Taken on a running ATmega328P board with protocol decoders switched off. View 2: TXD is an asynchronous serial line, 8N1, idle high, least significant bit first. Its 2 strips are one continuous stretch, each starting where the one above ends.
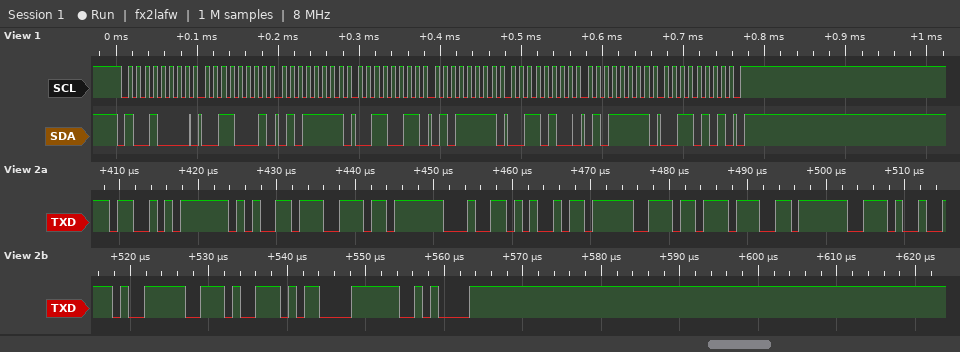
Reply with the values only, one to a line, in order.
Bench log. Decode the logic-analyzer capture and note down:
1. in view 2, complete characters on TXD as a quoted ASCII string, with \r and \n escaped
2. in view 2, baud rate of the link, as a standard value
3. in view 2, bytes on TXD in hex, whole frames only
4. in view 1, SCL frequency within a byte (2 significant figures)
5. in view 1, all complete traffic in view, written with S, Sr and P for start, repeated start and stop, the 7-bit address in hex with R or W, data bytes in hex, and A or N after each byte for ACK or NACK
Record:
"Sending...\r\n"
1000000 baud
0x53 0x65 0x6E 0x64 0x69 0x6E 0x67 0x2E 0x2E 0x2E 0x0D 0x0A
100 kHz
S 48W A 31 A 5F A 33 A 5F A 34 A 5F A 35 A P
